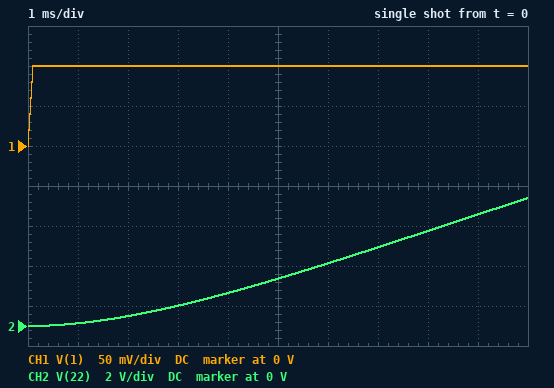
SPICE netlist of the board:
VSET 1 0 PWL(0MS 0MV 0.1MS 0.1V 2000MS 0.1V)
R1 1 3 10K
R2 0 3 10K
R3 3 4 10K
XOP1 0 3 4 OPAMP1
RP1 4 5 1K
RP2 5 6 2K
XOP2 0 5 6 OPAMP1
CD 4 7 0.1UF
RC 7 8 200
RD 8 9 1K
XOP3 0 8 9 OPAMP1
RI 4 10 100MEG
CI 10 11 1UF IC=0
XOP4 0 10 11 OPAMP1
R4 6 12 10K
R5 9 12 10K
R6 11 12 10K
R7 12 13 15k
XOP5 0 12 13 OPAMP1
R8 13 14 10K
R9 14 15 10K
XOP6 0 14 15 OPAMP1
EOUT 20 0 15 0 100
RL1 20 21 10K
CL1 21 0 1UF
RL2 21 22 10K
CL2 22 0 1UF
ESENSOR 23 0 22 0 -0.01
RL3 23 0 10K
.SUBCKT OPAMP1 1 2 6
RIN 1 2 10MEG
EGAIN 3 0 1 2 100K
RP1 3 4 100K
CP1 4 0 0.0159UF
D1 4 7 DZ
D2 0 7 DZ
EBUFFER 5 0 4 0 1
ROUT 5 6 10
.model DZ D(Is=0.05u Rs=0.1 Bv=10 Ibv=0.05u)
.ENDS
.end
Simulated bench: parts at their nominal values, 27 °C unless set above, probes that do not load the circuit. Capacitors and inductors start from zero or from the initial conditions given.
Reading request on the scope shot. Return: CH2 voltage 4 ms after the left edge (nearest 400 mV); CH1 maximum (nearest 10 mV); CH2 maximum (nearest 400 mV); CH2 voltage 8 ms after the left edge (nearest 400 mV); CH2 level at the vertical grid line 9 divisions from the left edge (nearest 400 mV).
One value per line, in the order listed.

1.6 V
100 mV
6.4 V
4.8 V
5.6 V
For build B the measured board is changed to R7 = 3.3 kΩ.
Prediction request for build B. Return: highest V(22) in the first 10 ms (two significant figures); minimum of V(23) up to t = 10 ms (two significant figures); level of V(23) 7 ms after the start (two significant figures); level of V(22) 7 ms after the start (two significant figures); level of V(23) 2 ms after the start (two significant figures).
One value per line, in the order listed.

1.4 V
-14 mV
-8.7 mV
870 mV
-1.1 mV
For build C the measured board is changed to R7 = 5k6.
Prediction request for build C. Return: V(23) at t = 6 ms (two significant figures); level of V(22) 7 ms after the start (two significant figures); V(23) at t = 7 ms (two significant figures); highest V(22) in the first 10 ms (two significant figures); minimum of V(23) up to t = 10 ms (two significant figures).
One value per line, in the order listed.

-12 mV
1.5 V
-15 mV
2.4 V
-24 mV
